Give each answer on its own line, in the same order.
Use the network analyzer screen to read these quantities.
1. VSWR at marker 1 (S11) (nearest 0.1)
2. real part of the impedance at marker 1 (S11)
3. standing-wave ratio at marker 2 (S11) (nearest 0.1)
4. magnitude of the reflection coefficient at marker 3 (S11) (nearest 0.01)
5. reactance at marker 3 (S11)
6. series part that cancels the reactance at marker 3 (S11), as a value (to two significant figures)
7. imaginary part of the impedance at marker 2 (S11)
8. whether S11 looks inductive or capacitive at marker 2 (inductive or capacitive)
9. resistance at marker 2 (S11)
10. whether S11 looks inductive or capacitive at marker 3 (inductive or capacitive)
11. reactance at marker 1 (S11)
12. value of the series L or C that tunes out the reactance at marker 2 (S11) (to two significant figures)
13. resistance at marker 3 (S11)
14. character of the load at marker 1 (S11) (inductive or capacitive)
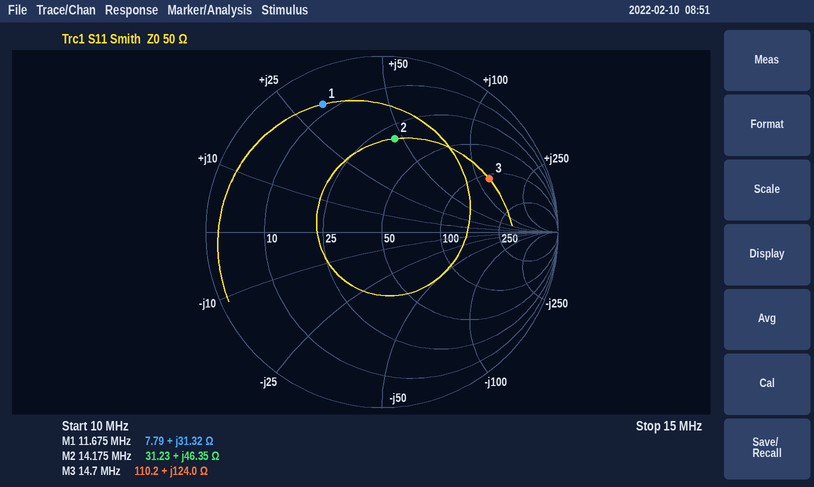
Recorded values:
9.0
7.79 Ω
3.3
0.68
+124.0 Ω
87 pF
+46.35 Ω
inductive
31.23 Ω
inductive
+31.32 Ω
240 pF
110.2 Ω
inductive
